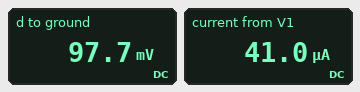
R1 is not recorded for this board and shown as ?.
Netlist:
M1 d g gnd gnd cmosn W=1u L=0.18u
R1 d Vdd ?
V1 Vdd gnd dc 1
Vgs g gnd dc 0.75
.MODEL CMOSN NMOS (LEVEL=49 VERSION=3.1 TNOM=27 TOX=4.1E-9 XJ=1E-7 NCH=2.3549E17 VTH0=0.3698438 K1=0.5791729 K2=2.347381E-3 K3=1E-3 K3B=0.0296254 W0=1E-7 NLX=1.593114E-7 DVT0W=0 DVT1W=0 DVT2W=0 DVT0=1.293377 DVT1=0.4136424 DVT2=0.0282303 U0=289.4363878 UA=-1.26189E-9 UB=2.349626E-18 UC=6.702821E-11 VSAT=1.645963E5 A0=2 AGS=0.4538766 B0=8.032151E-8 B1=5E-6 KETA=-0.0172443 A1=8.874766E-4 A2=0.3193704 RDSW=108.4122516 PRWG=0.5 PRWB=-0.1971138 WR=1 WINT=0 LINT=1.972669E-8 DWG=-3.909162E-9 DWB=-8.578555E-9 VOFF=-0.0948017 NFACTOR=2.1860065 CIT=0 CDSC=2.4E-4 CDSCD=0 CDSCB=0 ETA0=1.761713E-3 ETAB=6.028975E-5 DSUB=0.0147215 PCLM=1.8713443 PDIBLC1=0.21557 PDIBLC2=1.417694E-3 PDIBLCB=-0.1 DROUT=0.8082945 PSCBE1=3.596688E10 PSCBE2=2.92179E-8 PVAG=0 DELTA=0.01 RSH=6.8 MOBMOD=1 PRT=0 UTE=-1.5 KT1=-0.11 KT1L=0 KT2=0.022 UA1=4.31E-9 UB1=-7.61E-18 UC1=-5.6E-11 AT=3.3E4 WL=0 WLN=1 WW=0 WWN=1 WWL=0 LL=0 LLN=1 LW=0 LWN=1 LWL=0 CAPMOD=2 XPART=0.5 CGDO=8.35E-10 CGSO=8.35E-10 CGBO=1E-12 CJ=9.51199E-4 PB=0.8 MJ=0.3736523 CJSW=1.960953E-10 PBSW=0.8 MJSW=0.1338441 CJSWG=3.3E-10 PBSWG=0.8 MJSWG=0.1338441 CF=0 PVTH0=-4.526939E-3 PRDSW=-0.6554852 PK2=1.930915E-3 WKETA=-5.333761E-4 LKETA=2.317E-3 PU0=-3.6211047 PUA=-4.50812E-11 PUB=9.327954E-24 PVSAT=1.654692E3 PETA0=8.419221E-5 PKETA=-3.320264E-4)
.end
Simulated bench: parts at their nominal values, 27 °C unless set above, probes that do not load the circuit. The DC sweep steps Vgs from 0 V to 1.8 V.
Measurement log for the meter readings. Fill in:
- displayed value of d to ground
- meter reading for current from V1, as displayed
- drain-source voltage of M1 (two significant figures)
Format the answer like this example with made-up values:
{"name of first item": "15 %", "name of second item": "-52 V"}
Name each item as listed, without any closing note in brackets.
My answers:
{"displayed value of d to ground": "97.7 mV", "meter reading for current from V1, as displayed": "41.0 µA", "drain-source voltage of M1": "98 mV"}
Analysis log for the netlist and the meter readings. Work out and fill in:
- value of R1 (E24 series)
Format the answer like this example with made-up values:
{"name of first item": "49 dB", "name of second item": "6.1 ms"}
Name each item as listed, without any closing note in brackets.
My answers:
{"value of R1": "22 kΩ"}
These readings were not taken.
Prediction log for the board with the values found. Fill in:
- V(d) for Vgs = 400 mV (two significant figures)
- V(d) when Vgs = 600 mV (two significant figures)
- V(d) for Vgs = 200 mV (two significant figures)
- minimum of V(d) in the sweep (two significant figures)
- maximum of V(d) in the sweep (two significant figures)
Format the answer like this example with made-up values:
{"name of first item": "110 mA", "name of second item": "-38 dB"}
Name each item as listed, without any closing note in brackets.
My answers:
{"V(d) for Vgs = 400 mV": "980 mV", "V(d) when Vgs = 600 mV": "470 mV", "V(d) for Vgs = 200 mV": "1.0 V", "minimum of V(d) in the sweep": "27 mV", "maximum of V(d) in the sweep": "1.0 V"}
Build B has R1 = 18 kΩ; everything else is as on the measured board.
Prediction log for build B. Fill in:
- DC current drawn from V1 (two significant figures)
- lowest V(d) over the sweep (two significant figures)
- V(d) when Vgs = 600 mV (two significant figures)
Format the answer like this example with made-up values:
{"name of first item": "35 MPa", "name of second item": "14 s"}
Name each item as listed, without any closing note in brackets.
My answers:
{"DC current drawn from V1": "49 µA", "lowest V(d) over the sweep": "33 mV", "V(d) when Vgs = 600 mV": "550 mV"}
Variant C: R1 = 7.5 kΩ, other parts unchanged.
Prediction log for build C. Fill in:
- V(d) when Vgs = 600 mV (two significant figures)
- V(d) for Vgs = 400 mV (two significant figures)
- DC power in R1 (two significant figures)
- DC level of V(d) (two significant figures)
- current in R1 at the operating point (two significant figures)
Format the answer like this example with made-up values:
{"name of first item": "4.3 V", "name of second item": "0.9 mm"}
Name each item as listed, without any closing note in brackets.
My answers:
{"V(d) when Vgs = 600 mV": "790 mV", "V(d) for Vgs = 400 mV": "990 mV", "DC power in R1": "43 µW", "DC level of V(d)": "430 mV", "current in R1 at the operating point": "76 µA"}
